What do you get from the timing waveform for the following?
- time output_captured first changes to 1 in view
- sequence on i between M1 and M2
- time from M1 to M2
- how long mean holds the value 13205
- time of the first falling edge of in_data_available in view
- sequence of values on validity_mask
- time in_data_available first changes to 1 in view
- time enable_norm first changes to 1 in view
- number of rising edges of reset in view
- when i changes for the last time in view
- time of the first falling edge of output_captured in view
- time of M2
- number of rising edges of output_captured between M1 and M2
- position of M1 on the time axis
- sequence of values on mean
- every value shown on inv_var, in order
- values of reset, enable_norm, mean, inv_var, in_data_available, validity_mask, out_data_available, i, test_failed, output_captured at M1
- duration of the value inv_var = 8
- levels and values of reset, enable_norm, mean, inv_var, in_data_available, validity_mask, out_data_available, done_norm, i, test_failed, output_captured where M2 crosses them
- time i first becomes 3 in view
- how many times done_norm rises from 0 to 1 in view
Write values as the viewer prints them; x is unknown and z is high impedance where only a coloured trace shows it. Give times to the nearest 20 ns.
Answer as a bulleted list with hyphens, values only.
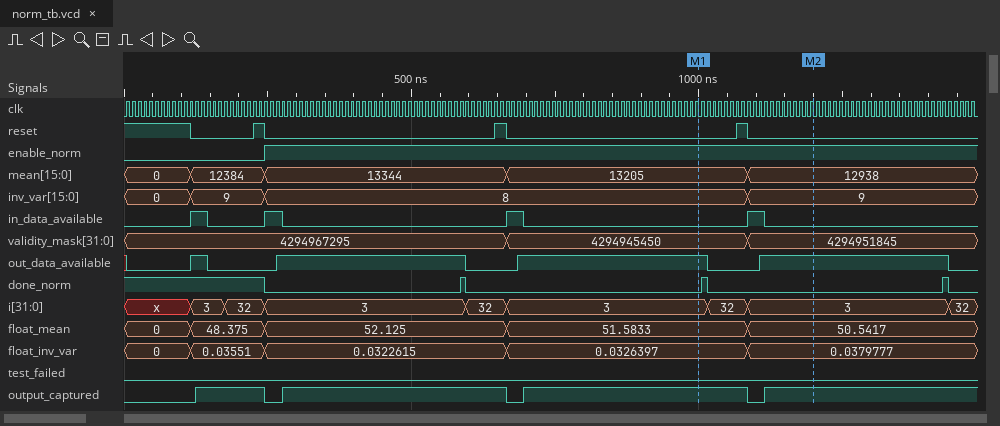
- 120 ns
- 3, 32, 3
- 200 ns
- 420 ns
- 140 ns
- 4294967295, 4294945450, 4294951845
- 120 ns
- 240 ns
- 3
- 1440 ns
- 240 ns
- 1200 ns
- 1
- 1000 ns
- 0, 12384, 13344, 13205, 12938
- 0, 9, 8, 9
- reset=0, enable_norm=1, mean=13205, inv_var=8, in_data_available=0, validity_mask=4294945450, out_data_available=1, i=3, test_failed=0, output_captured=1
- 840 ns
- reset=0, enable_norm=1, mean=12938, inv_var=9, in_data_available=0, validity_mask=4294951845, out_data_available=1, done_norm=0, i=3, test_failed=0, output_captured=1
- 120 ns
- 3
